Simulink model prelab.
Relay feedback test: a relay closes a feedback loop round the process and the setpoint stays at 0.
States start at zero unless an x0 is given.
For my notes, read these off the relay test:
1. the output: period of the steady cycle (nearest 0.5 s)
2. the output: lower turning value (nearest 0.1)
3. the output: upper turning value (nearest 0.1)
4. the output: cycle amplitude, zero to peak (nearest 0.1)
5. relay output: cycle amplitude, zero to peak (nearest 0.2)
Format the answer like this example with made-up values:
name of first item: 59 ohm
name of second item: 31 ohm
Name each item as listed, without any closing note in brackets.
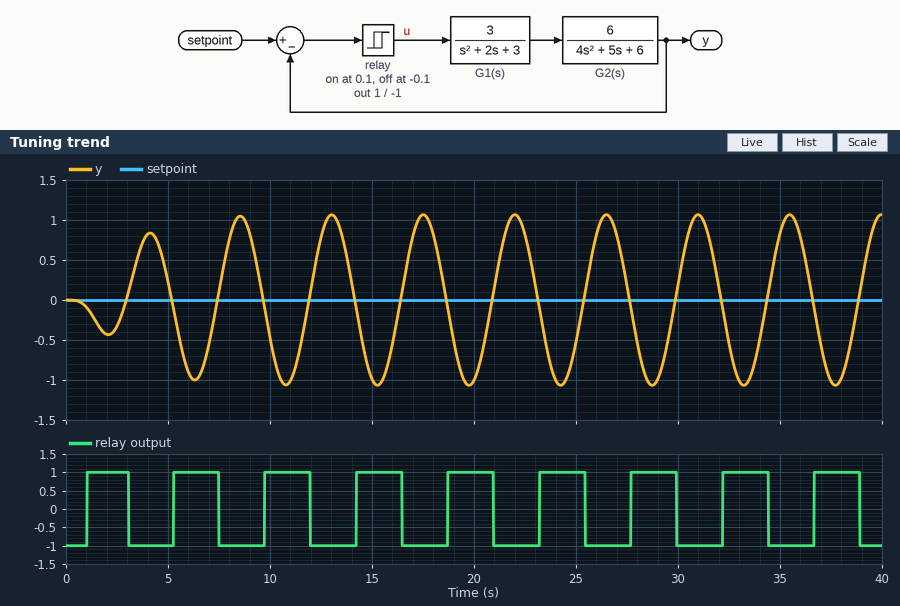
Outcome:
the output: period of the steady cycle: 4.5 s
the output: lower turning value: -1.1
the output: upper turning value: 1.1
the output: cycle amplitude, zero to peak: 1.1
relay output: cycle amplitude, zero to peak: 1.0
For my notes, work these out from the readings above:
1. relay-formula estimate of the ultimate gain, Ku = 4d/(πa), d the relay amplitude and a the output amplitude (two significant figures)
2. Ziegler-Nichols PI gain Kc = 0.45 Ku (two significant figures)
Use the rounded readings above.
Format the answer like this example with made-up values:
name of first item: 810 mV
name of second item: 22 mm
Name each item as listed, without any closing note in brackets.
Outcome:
relay-formula estimate of the ultimate gain, Ku = 4d/(πa), d the relay amplitude and a the output amplitude: 1.2
Ziegler-Nichols PI gain Kc = 0.45 Ku: 0.54
